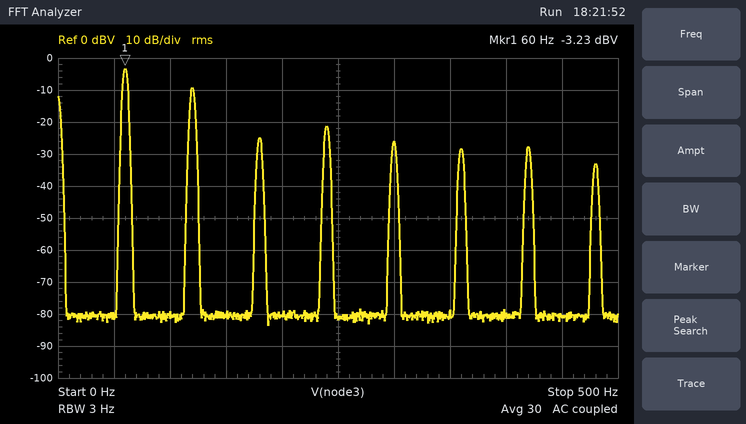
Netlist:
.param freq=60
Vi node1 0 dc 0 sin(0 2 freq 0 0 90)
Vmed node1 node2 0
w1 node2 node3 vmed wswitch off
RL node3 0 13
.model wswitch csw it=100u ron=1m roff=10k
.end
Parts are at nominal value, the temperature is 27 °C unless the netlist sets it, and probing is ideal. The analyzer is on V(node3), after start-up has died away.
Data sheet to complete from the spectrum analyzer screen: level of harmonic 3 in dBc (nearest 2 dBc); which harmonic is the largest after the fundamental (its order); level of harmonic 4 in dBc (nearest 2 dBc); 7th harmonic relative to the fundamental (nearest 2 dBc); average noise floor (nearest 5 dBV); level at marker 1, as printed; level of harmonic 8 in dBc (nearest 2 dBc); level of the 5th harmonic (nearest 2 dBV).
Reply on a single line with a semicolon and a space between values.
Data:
-22 dBc; 2; -18 dBc; -24 dBc; -80 dBV; -3.23 dBV; -30 dBc; -26 dBV
